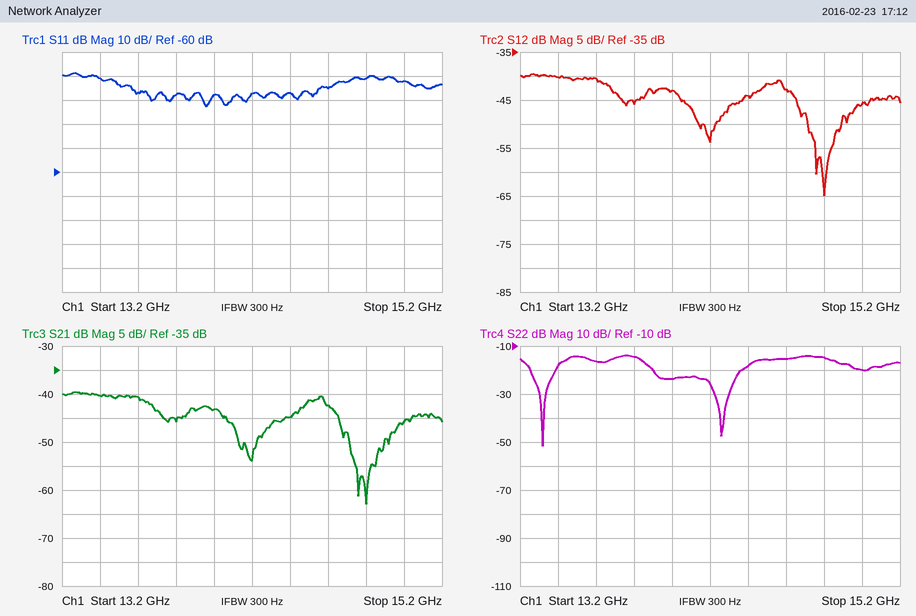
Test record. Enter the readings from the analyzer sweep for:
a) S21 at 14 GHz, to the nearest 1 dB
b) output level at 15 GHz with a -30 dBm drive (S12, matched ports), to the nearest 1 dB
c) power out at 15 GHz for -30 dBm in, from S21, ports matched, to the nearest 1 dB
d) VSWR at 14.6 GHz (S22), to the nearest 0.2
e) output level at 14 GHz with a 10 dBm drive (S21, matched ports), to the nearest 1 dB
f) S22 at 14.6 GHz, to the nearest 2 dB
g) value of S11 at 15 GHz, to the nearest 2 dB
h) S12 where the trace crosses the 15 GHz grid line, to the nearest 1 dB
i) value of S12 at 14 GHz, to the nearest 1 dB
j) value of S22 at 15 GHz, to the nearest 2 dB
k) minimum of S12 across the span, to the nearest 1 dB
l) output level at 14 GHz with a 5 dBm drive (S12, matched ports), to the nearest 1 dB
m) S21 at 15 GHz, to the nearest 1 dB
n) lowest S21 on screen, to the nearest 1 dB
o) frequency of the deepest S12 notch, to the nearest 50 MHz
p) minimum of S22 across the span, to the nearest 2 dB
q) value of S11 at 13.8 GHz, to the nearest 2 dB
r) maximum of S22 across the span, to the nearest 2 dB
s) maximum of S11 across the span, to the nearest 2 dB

-43 dB
-76 dBm
-76 dBm
1.4
-33 dBm
-16 dB
-22 dB
-46 dB
-43 dB
-20 dB
-65 dB
-38 dBm
-46 dB
-63 dB
14.80 GHz
-52 dB
-28 dB
-14 dB
-18 dB
